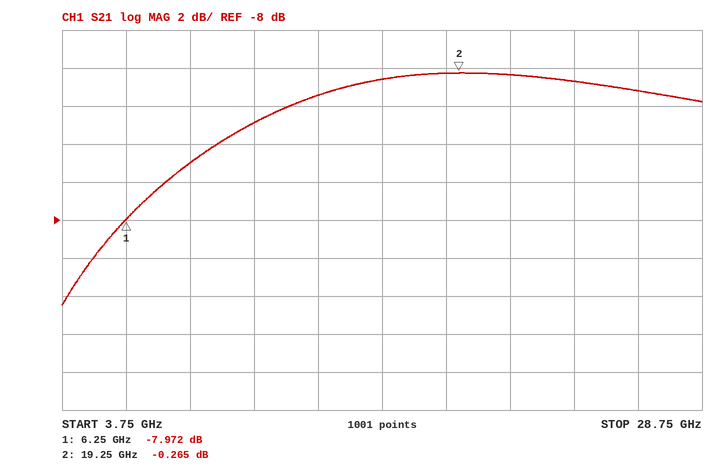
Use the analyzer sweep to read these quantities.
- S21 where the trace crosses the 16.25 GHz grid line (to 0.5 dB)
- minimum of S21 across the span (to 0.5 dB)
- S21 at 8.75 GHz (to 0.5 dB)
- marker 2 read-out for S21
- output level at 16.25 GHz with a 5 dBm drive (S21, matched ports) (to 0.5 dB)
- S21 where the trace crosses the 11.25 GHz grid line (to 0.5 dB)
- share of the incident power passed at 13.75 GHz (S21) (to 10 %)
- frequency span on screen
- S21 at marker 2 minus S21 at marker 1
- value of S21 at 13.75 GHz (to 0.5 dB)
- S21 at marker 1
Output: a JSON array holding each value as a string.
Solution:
["-0.5 dB", "-12.5 dB", "-5.0 dB", "-0.265 dB", "4.5 dBm", "-3.0 dB", "70 %", "25 GHz", "7.707 dB", "-1.5 dB", "-7.972 dB"]
